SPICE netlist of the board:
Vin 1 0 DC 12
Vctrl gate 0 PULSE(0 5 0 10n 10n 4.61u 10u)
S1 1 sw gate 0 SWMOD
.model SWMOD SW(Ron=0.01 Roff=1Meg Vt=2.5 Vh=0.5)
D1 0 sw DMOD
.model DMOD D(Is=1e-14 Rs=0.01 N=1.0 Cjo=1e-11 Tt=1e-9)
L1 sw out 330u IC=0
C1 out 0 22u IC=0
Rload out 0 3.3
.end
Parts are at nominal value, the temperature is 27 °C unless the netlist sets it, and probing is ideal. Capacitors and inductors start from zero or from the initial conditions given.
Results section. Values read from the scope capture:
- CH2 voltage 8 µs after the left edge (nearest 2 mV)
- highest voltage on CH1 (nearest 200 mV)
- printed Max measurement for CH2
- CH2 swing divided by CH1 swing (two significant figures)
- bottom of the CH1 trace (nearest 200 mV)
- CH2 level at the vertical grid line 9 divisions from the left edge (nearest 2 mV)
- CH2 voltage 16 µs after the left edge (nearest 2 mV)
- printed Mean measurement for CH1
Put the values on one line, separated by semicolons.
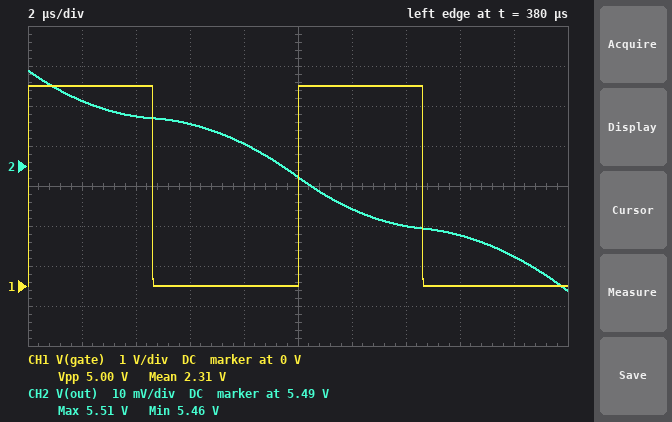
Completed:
5.496 V; 5.0 V; 5.51 V; 0.011; 0 V; 5.468 V; 5.472 V; 2.31 V
